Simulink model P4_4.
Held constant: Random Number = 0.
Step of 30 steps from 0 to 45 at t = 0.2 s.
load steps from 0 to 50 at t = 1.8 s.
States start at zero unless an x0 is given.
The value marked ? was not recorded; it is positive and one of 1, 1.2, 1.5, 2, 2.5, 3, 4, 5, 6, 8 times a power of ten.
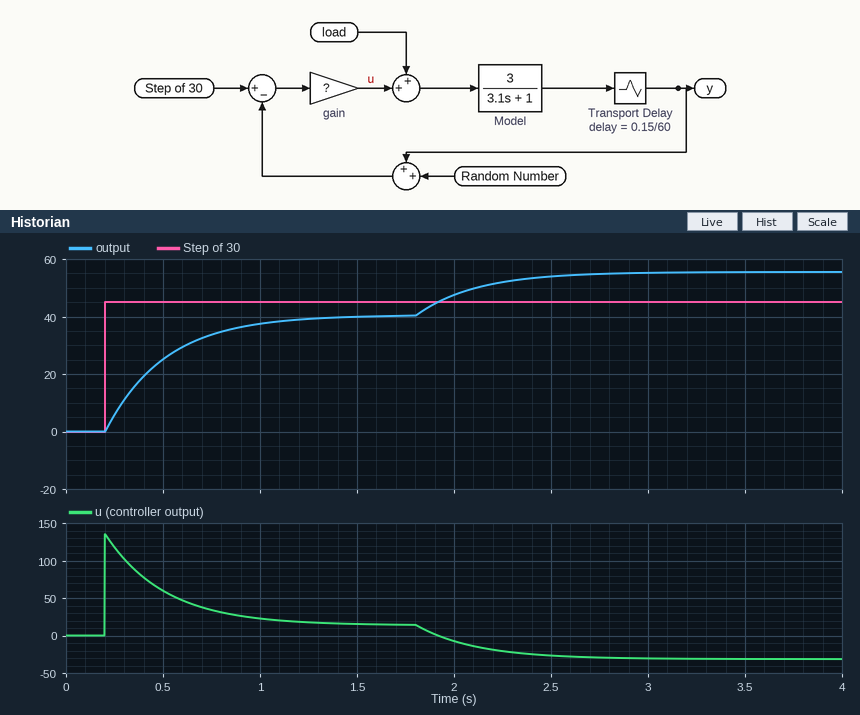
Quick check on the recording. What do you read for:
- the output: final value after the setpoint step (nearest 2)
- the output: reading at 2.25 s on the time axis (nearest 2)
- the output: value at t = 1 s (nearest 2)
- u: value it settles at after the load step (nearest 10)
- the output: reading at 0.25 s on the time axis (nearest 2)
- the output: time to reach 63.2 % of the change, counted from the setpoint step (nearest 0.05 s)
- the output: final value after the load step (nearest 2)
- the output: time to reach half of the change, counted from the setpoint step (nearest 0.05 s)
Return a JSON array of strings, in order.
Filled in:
["40", "52", "38", "-30", "6", "0.30 s", "56", "0.20 s"]
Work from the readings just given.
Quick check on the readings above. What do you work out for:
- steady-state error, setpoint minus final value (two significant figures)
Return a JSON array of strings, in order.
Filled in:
["5.0"]
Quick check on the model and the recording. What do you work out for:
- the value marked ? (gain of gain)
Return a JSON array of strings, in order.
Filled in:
["3"]
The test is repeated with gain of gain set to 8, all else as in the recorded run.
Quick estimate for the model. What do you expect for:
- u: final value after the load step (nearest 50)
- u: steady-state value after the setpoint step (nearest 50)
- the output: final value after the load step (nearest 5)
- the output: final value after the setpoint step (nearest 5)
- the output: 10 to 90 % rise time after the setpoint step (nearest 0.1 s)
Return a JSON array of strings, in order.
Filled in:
["-50", "0", "50", "45", "0.3 s"]
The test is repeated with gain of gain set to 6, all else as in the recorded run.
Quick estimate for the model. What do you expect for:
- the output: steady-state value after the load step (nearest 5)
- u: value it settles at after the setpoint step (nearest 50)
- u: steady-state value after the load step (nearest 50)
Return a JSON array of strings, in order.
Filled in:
["50", "0", "-50"]
